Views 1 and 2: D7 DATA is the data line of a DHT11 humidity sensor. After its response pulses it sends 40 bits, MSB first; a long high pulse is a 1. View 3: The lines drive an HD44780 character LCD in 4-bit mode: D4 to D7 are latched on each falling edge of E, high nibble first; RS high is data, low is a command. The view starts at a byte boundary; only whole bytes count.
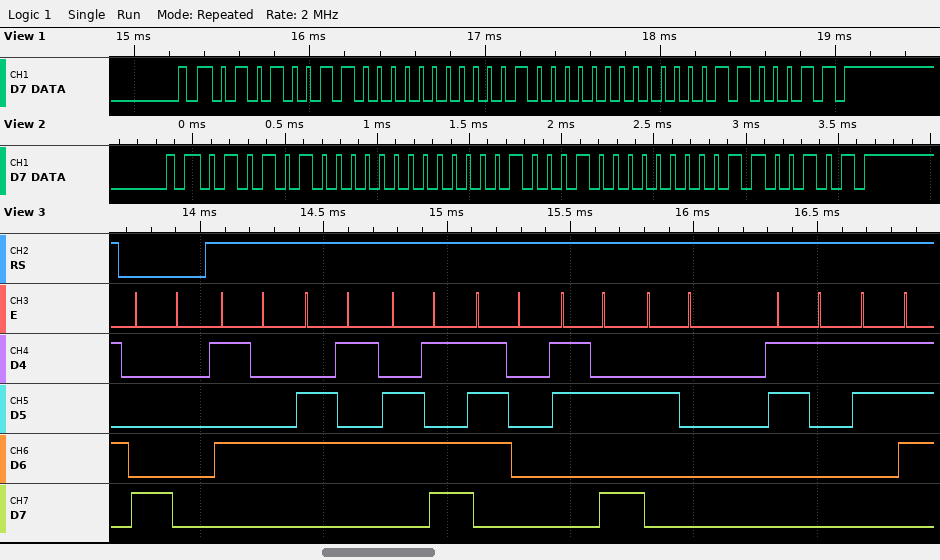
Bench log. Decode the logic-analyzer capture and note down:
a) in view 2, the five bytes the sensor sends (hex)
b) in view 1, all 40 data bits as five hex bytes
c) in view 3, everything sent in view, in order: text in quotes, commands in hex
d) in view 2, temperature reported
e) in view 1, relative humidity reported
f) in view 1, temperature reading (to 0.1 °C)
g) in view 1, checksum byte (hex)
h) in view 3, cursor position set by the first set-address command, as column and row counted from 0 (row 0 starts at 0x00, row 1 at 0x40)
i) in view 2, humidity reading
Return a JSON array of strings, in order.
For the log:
["54 00 11 00 65", "53 00 10 00 63", "0x80 \"Temp: 17\"", "17.0 °C", "83 %", "16.0 °C", "0x63", "column 0, row 0", "84 %"]
